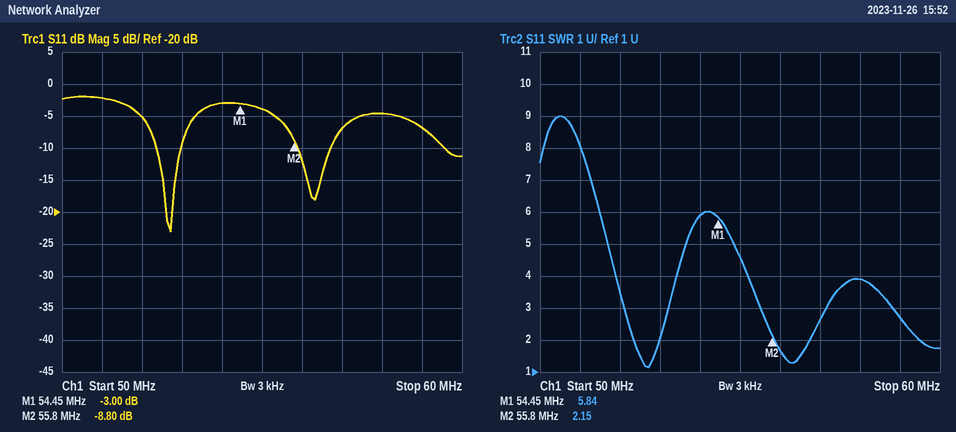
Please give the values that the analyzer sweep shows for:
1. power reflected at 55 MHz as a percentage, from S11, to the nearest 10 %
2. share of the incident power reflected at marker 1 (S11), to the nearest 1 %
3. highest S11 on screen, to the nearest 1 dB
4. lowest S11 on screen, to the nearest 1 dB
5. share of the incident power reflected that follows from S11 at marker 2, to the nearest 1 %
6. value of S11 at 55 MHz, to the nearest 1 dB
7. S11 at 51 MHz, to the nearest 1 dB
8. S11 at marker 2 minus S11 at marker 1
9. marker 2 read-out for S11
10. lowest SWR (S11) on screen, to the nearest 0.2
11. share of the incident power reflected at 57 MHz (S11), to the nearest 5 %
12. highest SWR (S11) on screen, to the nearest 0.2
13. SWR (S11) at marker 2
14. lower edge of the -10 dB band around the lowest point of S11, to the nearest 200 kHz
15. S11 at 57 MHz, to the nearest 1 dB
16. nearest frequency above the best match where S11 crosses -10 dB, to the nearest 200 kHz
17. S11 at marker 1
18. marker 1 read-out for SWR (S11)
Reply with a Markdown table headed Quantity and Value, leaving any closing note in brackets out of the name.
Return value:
| Quantity | Value |
|---|---|
| power reflected at 55 MHz as a percentage, from S11, to the nearest 10 % | 40 % |
| share of the incident power reflected at marker 1 (S11), to the nearest 1 % | 50 % |
| highest S11 on screen, to the nearest 1 dB | -2 dB |
| lowest S11 on screen, to the nearest 1 dB | -23 dB |
| share of the incident power reflected that follows from S11 at marker 2, to the nearest 1 % | 13 % |
| value of S11 at 55 MHz, to the nearest 1 dB | -4 dB |
| S11 at 51 MHz, to the nearest 1 dB | -2 dB |
| S11 at marker 2 minus S11 at marker 1 | -5.80 dB |
| marker 2 read-out for S11 | -8.80 dB |
| lowest SWR (S11) on screen, to the nearest 0.2 | 1.2 |
| share of the incident power reflected at 57 MHz (S11), to the nearest 5 % | 20 % |
| highest SWR (S11) on screen, to the nearest 0.2 | 9.0 |
| SWR (S11) at marker 2 | 2.15 |
| lower edge of the -10 dB band around the lowest point of S11, to the nearest 200 kHz | 52.4 MHz |
| S11 at 57 MHz, to the nearest 1 dB | -7 dB |
| nearest frequency above the best match where S11 crosses -10 dB, to the nearest 200 kHz | 53.0 MHz |
| S11 at marker 1 | -3.00 dB |
| marker 1 read-out for SWR | 5.84 |
